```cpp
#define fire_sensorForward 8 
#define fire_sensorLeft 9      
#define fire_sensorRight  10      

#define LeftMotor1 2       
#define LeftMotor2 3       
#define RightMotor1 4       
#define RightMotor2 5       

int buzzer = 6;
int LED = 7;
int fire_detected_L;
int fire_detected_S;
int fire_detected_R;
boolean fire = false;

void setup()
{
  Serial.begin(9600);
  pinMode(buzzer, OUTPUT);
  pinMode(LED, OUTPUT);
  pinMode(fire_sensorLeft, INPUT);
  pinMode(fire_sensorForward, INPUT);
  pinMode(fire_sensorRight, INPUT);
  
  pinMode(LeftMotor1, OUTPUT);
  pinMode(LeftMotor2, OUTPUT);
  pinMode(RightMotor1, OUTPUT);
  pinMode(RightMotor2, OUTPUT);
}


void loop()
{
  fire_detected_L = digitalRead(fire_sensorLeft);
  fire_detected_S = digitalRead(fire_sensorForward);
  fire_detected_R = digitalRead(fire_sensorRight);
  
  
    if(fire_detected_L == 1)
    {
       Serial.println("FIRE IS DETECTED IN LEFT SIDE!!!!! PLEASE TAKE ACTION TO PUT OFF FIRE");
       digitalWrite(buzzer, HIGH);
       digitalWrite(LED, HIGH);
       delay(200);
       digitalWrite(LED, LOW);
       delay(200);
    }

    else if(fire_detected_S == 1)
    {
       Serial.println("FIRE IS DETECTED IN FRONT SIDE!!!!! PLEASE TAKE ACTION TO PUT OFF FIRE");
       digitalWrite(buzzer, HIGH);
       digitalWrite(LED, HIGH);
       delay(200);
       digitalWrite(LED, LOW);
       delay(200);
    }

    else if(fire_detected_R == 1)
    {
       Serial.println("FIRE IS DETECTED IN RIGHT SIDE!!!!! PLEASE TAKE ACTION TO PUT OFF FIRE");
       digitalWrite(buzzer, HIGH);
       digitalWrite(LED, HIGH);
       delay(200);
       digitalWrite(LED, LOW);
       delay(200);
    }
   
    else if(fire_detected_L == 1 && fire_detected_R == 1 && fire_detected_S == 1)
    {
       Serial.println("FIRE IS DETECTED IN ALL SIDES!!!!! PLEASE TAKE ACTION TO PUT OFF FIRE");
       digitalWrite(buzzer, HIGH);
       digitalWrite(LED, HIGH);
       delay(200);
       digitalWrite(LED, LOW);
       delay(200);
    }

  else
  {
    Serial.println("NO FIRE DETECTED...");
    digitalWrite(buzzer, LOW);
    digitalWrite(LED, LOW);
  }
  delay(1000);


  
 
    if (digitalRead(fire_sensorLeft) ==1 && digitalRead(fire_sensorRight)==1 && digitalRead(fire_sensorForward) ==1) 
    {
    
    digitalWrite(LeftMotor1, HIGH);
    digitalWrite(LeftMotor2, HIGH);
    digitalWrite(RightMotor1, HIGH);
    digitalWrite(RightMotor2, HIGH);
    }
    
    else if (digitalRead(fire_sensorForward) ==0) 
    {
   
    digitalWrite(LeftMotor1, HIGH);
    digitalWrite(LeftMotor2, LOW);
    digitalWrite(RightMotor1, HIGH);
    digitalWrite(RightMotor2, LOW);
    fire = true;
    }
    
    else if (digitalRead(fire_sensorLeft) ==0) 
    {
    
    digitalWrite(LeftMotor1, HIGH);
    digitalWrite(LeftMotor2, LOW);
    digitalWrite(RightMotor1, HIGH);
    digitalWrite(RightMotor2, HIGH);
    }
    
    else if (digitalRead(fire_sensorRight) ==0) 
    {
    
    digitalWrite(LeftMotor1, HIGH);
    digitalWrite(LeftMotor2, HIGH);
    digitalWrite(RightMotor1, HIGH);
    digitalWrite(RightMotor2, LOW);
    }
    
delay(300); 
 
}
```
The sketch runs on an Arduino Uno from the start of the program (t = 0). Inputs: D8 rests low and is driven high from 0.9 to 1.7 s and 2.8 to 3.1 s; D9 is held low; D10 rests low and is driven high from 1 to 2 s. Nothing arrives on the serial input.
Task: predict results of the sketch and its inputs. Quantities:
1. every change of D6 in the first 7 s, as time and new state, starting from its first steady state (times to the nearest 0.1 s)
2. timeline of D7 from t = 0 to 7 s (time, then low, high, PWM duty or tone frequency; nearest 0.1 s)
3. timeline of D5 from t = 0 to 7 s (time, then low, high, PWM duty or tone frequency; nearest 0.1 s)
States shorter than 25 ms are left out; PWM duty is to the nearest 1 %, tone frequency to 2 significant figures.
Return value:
0 s low; 1.3 s high; 4.7 s low
0 s low; 1.3 s high; 1.5 s low; 3 s high; 3.2 s low
0 s low; 1 s high; 2.7 s low
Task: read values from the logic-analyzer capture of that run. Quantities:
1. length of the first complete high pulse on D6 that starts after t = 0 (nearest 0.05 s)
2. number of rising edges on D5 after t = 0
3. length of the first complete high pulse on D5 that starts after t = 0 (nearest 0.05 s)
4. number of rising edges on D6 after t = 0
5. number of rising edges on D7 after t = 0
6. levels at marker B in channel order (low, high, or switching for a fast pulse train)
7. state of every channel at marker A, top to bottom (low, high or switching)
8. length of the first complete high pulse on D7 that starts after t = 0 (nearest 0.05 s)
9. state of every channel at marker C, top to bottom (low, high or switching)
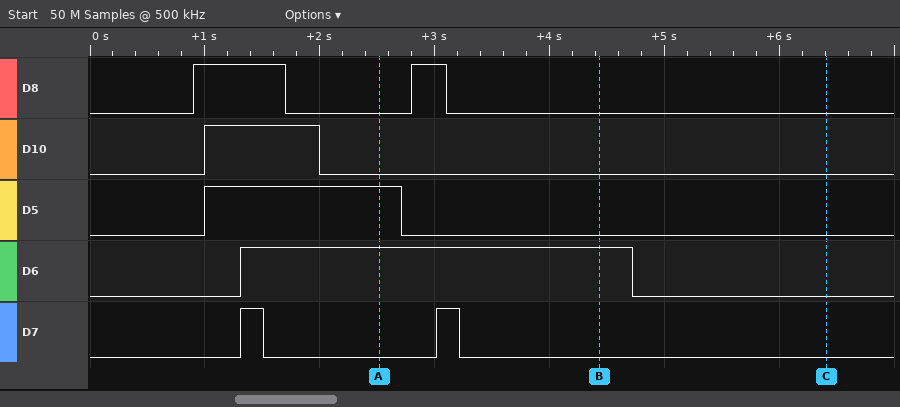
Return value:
3.40 s
1
1.70 s
1
2
D8 low, D10 low, D5 low, D6 high, D7 low
D8 low, D10 low, D5 high, D6 high, D7 low
0.20 s
D8 low, D10 low, D5 low, D6 low, D7 low
